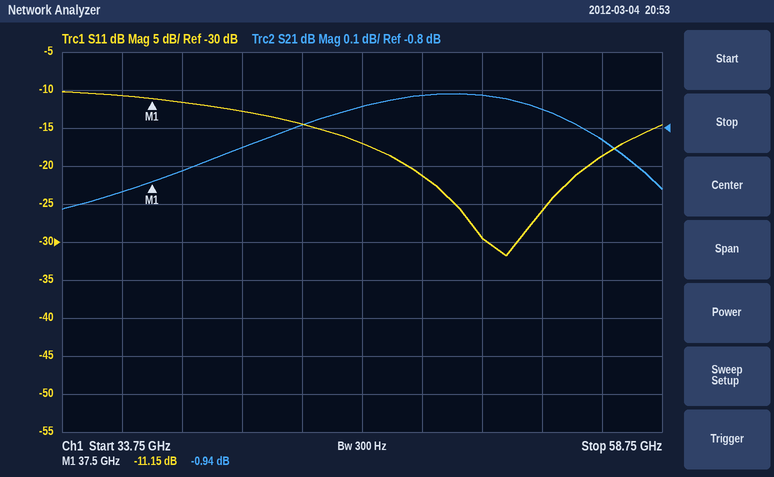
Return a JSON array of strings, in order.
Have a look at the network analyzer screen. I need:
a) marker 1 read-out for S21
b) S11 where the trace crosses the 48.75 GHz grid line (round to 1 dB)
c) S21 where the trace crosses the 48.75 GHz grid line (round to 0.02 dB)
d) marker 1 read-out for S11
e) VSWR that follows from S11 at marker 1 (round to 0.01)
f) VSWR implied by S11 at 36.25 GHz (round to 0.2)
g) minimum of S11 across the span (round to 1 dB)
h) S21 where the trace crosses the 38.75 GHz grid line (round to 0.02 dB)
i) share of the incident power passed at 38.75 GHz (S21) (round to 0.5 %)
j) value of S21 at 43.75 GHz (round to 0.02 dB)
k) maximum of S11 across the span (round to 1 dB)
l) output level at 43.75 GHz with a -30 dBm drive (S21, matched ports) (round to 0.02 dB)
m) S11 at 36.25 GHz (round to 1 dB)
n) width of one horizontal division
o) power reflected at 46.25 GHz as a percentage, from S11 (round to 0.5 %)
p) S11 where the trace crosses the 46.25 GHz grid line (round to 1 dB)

["-0.94 dB", "-21 dB", "-0.72 dB", "-11.15 dB", "1.77", "1.8", "-32 dB", "-0.92 dB", "81.0 %", "-0.80 dB", "-10 dB", "-30.80 dBm", "-11 dB", "2.5 GHz", "2.0 %", "-17 dB"]
